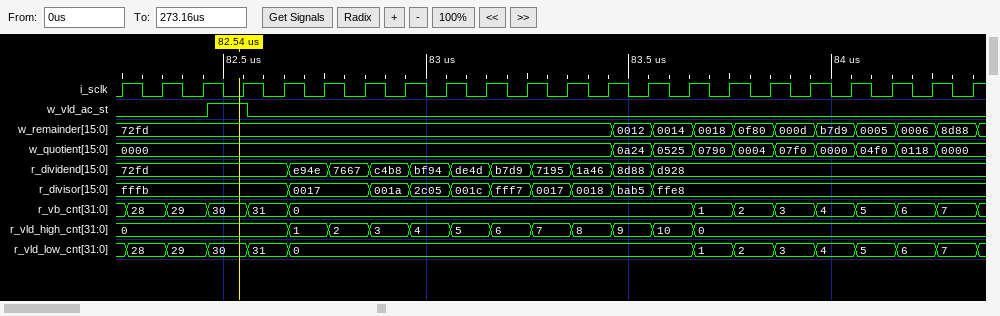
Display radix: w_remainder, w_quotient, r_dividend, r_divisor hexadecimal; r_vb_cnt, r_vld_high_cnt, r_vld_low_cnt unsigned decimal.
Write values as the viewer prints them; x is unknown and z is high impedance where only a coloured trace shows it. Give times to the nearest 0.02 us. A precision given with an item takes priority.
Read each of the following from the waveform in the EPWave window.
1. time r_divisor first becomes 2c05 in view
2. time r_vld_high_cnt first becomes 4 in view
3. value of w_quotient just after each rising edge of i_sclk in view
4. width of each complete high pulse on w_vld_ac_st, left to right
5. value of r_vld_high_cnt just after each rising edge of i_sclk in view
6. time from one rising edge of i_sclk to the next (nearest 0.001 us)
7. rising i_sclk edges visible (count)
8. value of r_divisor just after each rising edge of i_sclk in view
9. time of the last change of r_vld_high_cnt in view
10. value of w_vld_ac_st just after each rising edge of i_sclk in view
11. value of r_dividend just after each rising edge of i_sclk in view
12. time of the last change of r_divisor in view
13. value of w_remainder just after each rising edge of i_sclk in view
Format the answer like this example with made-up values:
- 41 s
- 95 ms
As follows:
- 82.96 us
- 82.96 us
- 0000, 0000, 0000, 0000, 0000, 0000, 0000, 0000, 0000, 0000, 0000, 0000, 0000, 0a24, 0525, 0790, 0004, 07f0, 0000, 04f0, 0118, 0000
- 0.1 us
- 0, 0, 0, 0, 0, 1, 2, 3, 4, 5, 6, 7, 8, 9, 10, 0, 0, 0, 0, 0, 0, 0
- 0.1 us
- 22
- fffb, fffb, fffb, fffb, fffb, 0017, 0017, 001a, 2c05, 001c, fff7, 0017, 0018, bab5, ffe8, ffe8, ffe8, ffe8, ffe8, ffe8, ffe8, ffe8
- 83.66 us
- 0 0 0 1 0 0 0 0 0 0 0 0 0 0 0 0 0 0 0 0 0 0
- 72fd, 72fd, 72fd, 72fd, 72fd, e94e, 7667, c4b8, bf94, de4d, b7d9, 7195, 1a46, 8d88, d928, d928, d928, d928, d928, d928, d928, d928
- 83.56 us
- 72fd, 72fd, 72fd, 72fd, 72fd, 72fd, 72fd, 72fd, 72fd, 72fd, 72fd, 72fd, 72fd, 0012, 0014, 0018, 0f80, 000d, b7d9, 0005, 0006, 8d88
